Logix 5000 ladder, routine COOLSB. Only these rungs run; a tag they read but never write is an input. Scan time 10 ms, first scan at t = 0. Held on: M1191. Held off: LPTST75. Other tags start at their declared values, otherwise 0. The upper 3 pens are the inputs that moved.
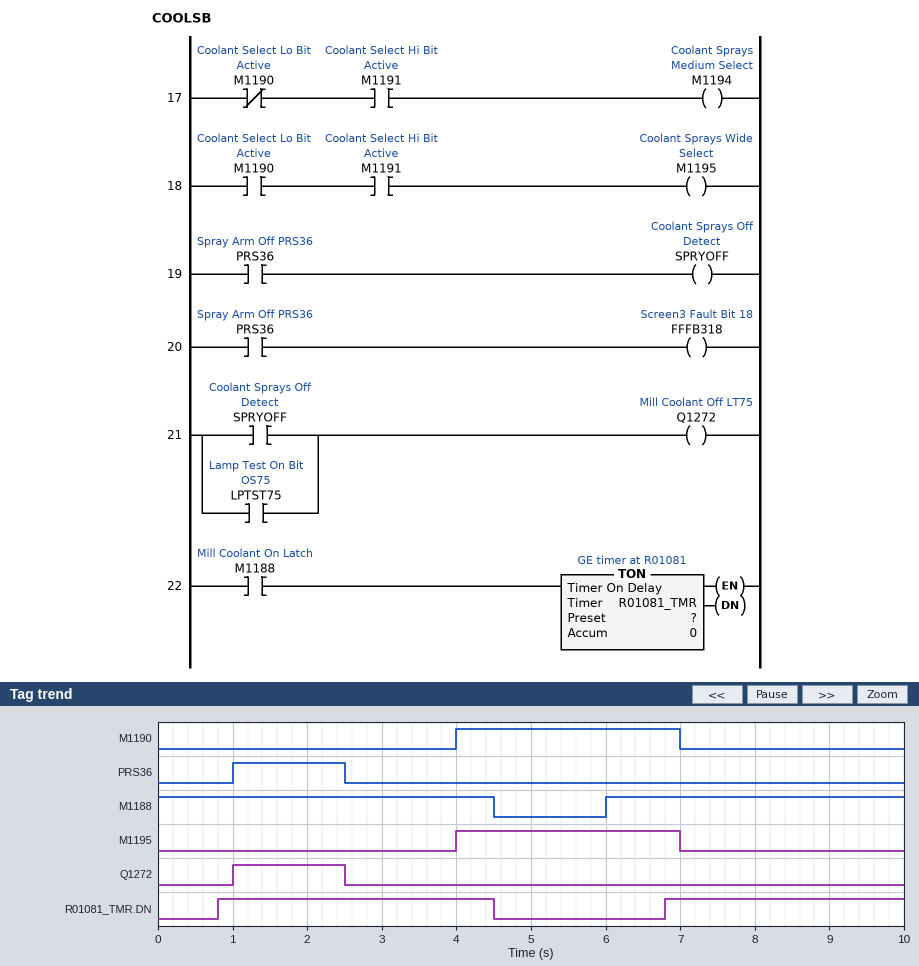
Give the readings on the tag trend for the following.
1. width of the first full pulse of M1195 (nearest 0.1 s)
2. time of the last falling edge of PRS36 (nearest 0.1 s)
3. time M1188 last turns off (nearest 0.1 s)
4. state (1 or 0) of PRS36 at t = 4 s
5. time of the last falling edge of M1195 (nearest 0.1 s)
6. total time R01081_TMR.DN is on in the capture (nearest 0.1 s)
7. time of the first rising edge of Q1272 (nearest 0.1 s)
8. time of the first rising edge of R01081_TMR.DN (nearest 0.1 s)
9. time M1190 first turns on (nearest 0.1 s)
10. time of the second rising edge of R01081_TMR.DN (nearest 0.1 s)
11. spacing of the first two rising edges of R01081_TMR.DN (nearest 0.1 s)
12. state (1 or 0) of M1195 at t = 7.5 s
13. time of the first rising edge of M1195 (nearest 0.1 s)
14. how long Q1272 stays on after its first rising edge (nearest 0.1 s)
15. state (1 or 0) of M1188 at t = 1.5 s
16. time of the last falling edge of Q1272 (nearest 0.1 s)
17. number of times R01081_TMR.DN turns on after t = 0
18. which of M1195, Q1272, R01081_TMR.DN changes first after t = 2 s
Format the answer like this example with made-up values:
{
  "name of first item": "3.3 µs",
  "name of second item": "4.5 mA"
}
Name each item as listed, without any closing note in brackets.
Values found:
{
  "width of the first full pulse of M1195": "3.0 s",
  "time of the last falling edge of PRS36": "2.5 s",
  "time M1188 last turns off": "4.5 s",
  "state (1 or 0) of PRS36 at t = 4 s": "0",
  "time of the last falling edge of M1195": "7.0 s",
  "total time R01081_TMR.DN is on in the capture": "6.9 s",
  "time of the first rising edge of Q1272": "1.0 s",
  "time of the first rising edge of R01081_TMR.DN": "0.8 s",
  "time M1190 first turns on": "4.0 s",
  "time of the second rising edge of R01081_TMR.DN": "6.8 s",
  "spacing of the first two rising edges of R01081_TMR.DN": "6.0 s",
  "state (1 or 0) of M1195 at t = 7.5 s": "0",
  "time of the first rising edge of M1195": "4.0 s",
  "how long Q1272 stays on after its first rising edge": "1.5 s",
  "state (1 or 0) of M1188 at t = 1.5 s": "1",
  "time of the last falling edge of Q1272": "2.5 s",
  "number of times R01081_TMR.DN turns on after t = 0": "2",
  "which of M1195, Q1272, R01081_TMR.DN changes first after t = 2 s": "Q1272"
}
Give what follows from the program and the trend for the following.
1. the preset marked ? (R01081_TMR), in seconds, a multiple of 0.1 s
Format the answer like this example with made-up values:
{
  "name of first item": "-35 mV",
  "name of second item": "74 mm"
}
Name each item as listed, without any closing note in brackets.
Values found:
{
  "the preset marked ? (R01081_TMR), in seconds, a multiple of 0.1 s": "0.8 s"
}
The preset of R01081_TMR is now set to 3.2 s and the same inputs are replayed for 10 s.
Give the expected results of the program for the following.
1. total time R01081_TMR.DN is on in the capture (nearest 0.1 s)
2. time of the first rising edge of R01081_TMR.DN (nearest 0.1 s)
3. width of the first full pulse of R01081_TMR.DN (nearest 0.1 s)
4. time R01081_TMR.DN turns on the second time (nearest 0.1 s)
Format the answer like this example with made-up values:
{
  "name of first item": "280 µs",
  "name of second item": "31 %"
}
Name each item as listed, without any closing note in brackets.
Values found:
{
  "total time R01081_TMR.DN is on in the capture": "2.1 s",
  "time of the first rising edge of R01081_TMR.DN": "3.2 s",
  "width of the first full pulse of R01081_TMR.DN": "1.3 s",
  "time R01081_TMR.DN turns on the second time": "9.2 s"
}
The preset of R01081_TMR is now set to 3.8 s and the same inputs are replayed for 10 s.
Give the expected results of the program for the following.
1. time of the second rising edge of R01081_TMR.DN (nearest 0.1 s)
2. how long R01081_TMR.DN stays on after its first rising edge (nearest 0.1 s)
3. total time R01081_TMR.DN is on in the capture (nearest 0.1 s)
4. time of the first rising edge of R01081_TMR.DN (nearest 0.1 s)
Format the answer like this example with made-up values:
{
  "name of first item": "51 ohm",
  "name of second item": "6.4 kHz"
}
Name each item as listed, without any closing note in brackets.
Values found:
{
  "time of the second rising edge of R01081_TMR.DN": "9.8 s",
  "how long R01081_TMR.DN stays on after its first rising edge": "0.7 s",
  "total time R01081_TMR.DN is on in the capture": "0.9 s",
  "time of the first rising edge of R01081_TMR.DN": "3.8 s"
}
